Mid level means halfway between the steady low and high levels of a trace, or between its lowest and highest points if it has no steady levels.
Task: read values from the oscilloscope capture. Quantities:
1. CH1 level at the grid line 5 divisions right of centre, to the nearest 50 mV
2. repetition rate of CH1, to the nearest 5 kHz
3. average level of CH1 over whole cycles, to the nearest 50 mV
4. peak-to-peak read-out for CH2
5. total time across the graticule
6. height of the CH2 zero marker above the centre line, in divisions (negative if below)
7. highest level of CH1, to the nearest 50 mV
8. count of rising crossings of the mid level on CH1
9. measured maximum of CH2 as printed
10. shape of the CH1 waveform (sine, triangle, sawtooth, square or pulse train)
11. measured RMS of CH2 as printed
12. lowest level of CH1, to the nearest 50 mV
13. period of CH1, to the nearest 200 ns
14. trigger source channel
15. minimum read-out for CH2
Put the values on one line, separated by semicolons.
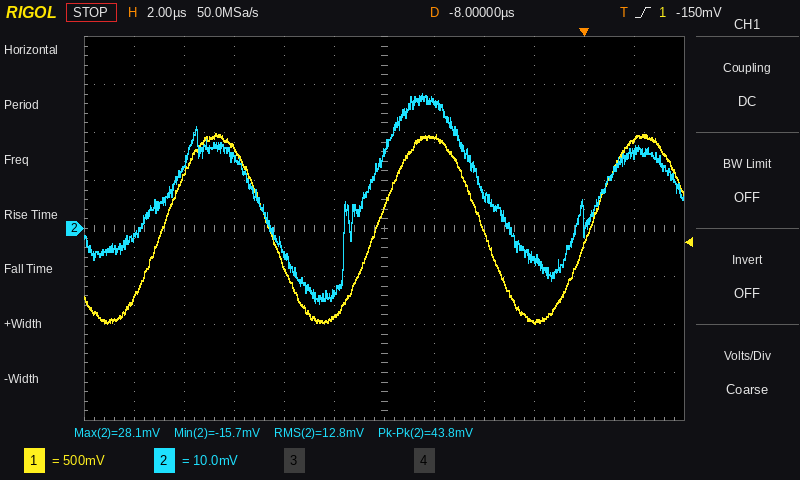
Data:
950 mV; 115 kHz; 0 mV; 43.8 mV; 24 µs; 0.0 div; 1.00 V; 3; 28.1 mV; sine; 12.8 mV; -1.00 V; 8.6 µs; CH1; -15.7 mV
